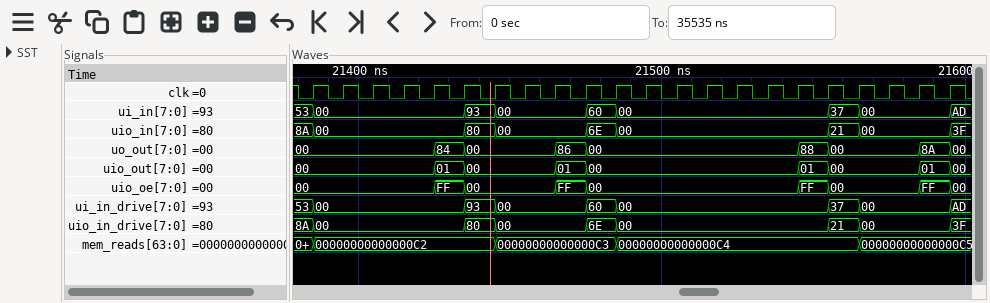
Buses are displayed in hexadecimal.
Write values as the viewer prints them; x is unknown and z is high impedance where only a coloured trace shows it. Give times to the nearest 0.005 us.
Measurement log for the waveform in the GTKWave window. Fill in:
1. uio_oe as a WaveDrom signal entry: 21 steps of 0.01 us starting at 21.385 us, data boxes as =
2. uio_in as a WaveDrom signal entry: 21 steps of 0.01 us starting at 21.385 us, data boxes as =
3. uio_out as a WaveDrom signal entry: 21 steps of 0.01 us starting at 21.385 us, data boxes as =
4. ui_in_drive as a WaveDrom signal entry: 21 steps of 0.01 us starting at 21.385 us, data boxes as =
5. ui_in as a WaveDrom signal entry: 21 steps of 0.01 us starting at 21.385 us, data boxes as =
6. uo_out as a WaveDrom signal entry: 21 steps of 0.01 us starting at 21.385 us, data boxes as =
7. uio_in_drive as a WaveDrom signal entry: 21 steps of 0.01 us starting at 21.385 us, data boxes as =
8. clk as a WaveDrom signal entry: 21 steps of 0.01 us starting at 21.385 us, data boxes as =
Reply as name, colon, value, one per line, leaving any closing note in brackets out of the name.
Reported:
uio_oe as a WaveDrom signal entry: 21 steps of 0.01 us starting at 21.385 us, data boxes as =: {name: 'uio_oe', wave: '=...==..==......==..=', data: '00 FF 00 FF 00 FF 00 FF'}
uio_in as a WaveDrom signal entry: 21 steps of 0.01 us starting at 21.385 us, data boxes as =: {name: 'uio_in', wave: '=....==..==......==..', data: '00 80 00 6E 00 21 00'}
uio_out as a WaveDrom signal entry: 21 steps of 0.01 us starting at 21.385 us, data boxes as =: {name: 'uio_out', wave: '=...==..==......==..=', data: '00 01 00 01 00 01 00 01'}
ui_in_drive as a WaveDrom signal entry: 21 steps of 0.01 us starting at 21.385 us, data boxes as =: {name: 'ui_in_drive', wave: '=....==..==......==..', data: '00 93 00 60 00 37 00'}
ui_in as a WaveDrom signal entry: 21 steps of 0.01 us starting at 21.385 us, data boxes as =: {name: 'ui_in', wave: '=....==..==......==..', data: '00 93 00 60 00 37 00'}
uo_out as a WaveDrom signal entry: 21 steps of 0.01 us starting at 21.385 us, data boxes as =: {name: 'uo_out', wave: '=...==..==......==..=', data: '00 84 00 86 00 88 00 8A'}
uio_in_drive as a WaveDrom signal entry: 21 steps of 0.01 us starting at 21.385 us, data boxes as =: {name: 'uio_in_drive', wave: '=....==..==......==..', data: '00 80 00 6E 00 21 00'}
clk as a WaveDrom signal entry: 21 steps of 0.01 us starting at 21.385 us, data boxes as =: {name: 'clk', wave: 'p....................'}
